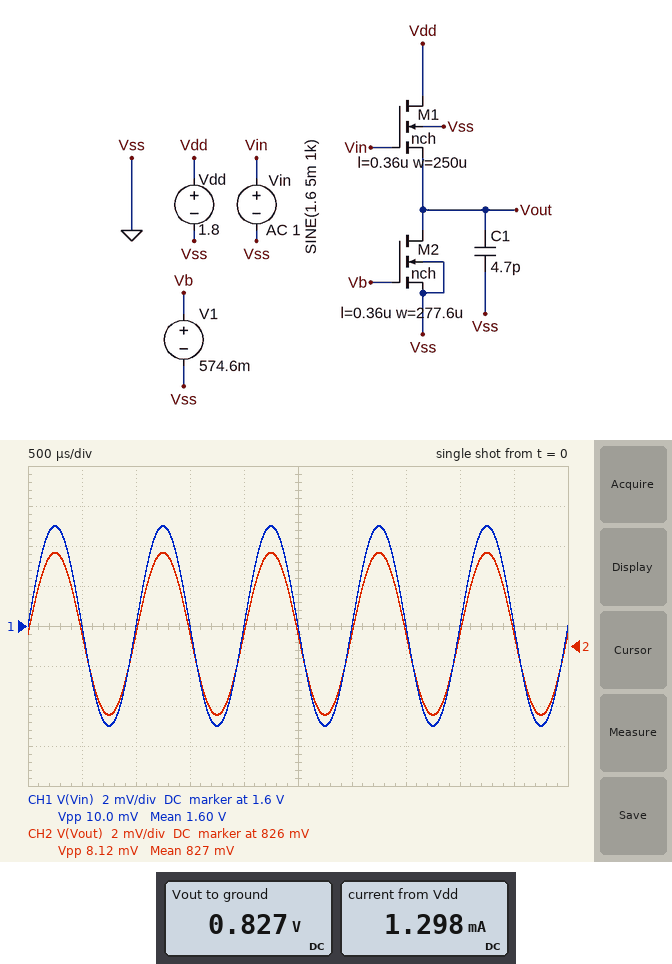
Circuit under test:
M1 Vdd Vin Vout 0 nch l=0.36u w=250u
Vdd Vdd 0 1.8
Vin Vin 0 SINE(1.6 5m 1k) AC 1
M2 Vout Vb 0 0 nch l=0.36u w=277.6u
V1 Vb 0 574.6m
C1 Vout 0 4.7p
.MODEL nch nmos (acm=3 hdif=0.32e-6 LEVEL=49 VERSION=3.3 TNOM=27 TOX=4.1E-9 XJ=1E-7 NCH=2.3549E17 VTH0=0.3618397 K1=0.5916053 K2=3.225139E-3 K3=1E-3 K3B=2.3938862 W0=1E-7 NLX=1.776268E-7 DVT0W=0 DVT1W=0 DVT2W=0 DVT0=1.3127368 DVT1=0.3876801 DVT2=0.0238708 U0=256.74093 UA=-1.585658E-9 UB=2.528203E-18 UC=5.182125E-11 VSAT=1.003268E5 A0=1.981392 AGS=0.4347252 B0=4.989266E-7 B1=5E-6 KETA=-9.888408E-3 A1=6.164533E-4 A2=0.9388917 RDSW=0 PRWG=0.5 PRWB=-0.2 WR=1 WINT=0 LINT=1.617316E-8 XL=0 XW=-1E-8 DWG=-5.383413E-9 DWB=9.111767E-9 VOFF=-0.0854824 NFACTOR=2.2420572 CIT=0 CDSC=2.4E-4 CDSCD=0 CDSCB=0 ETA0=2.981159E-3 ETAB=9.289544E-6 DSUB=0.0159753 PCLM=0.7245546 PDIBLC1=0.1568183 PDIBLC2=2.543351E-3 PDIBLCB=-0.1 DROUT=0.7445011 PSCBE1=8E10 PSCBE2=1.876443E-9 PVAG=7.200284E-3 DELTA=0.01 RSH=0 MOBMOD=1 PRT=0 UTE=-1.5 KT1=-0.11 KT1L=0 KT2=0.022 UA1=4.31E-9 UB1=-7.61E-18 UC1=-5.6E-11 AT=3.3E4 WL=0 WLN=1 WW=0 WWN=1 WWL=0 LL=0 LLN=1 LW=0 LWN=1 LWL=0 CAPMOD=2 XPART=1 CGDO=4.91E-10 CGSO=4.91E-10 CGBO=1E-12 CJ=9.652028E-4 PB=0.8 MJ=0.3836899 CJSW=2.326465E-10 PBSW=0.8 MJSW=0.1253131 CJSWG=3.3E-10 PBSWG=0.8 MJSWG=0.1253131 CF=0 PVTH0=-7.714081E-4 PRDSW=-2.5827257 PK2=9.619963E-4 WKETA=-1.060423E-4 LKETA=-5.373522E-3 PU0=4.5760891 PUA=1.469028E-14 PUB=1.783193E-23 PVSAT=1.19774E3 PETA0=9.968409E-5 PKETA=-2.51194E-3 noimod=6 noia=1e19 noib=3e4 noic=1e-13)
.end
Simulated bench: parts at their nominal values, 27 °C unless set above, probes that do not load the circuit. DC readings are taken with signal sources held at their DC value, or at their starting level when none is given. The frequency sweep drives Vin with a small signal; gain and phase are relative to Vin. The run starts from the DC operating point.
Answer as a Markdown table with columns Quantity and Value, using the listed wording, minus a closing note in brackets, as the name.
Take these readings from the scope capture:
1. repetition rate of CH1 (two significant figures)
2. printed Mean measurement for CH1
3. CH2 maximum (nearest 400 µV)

| Quantity | Value |
|---|---|
| repetition rate of CH1 | 1.0 kHz |
| printed Mean measurement for CH1 | 1.60 V |
| CH2 maximum | 830.8 mV |
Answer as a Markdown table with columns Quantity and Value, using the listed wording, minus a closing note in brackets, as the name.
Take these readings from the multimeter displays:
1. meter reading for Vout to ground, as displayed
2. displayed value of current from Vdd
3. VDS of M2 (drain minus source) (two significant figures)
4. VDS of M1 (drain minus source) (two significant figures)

| Quantity | Value |
|---|---|
| meter reading for Vout to ground, as displayed | 0.827 V |
| displayed value of current from Vdd | 1.298 mA |
| VDS of M2 (drain minus source) | 830 mV |
| VDS of M1 (drain minus source) | 970 mV |
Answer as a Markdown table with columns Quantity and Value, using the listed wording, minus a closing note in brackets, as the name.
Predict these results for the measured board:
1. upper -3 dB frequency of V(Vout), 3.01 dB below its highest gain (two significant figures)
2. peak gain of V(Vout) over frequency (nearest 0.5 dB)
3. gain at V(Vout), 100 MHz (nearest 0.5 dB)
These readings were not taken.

| Quantity | Value |
|---|---|
| upper -3 dB frequency of V(Vout), 3.01 dB below its highest gain | 670 MHz |
| peak gain of V(Vout) over frequency | -2.0 dB |
| gain at V(Vout), 100 MHz | -2.0 dB |
